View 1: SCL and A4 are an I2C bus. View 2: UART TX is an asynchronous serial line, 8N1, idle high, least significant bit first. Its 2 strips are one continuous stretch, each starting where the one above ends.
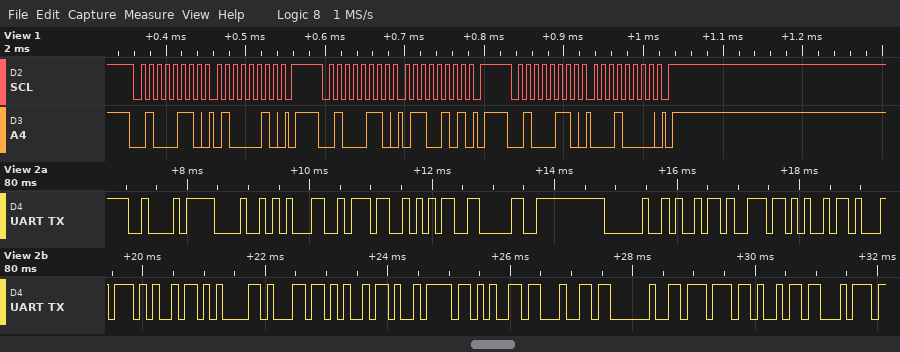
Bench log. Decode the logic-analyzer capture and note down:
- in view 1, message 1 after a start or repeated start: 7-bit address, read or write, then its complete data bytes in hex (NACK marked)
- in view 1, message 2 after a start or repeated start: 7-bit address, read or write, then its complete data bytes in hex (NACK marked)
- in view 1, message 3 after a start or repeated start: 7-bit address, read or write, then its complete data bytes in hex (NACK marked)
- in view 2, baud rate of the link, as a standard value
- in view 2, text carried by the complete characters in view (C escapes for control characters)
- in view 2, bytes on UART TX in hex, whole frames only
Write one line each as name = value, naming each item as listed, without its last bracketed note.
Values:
in view 1, message 1 after a start or repeated start: 7-bit address, read or write, then its complete data bytes in hex = 0x23 write: 42
in view 1, message 2 after a start or repeated start: 7-bit address, read or write, then its complete data bytes in hex = 0x23 write: 65
in view 1, message 3 after a start or repeated start: 7-bit address, read or write, then its complete data bytes in hex = 0x23 write: 10
in view 2, baud rate of the link, as a standard value = 9600 baud
in view 2, text carried by the complete characters in view = "BH1750 initialized wit"
in view 2, bytes on UART TX in hex, whole frames only = 42 48 31 37 35 30 20 69 6E 69 74 69 61 6C 69 7A 65 64 20 77 69 74
